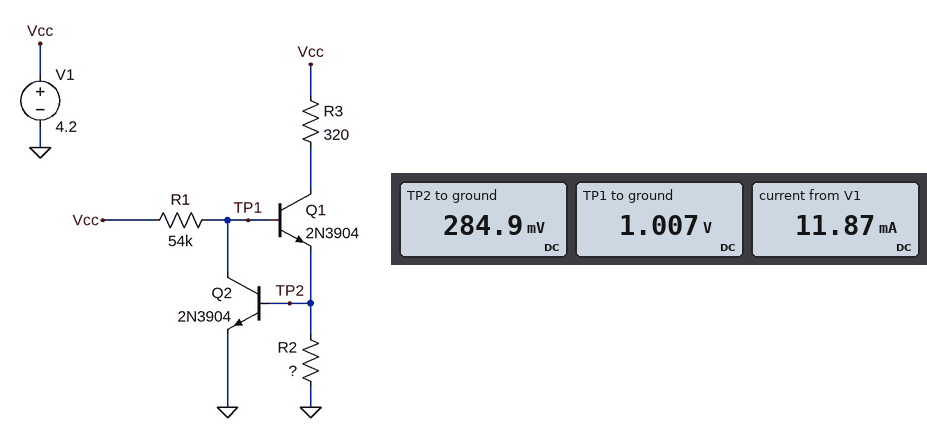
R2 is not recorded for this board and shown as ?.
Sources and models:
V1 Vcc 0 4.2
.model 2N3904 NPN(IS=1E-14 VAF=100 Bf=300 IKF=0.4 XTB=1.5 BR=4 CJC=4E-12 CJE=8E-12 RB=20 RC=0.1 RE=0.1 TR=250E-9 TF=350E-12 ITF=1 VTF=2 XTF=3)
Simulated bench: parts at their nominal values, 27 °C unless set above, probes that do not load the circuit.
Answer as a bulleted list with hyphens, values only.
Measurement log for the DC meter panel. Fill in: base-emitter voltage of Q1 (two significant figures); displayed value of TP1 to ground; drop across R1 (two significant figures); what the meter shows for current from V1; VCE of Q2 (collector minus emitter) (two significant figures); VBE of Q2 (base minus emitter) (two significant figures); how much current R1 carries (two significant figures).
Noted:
- 720 mV
- 1.007 V
- 3.2 V
- 11.87 mA
- 1.0 V
- 280 mV
- 59 µA
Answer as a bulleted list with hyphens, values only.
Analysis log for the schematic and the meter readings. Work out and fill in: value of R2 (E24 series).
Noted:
- 24 Ω
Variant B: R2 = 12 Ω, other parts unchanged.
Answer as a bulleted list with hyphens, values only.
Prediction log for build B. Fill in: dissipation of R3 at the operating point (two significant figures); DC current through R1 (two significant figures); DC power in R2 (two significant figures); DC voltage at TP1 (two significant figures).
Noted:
- 48 mW
- 62 µA
- 1.8 mW
- 870 mV
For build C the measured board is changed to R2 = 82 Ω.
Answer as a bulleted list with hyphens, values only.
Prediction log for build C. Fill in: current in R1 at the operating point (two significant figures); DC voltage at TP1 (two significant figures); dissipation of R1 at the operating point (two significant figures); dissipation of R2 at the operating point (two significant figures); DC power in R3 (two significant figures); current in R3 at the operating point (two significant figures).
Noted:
- 54 µA
- 1.3 V
- 160 µW
- 3.9 mW
- 15 mW
- 6.9 mA
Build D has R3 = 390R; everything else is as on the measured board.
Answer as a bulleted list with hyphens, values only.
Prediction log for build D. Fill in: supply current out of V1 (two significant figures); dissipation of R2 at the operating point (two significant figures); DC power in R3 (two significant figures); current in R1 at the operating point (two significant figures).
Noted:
- 9.9 mA
- 2.4 mW
- 38 mW
- 60 µA
